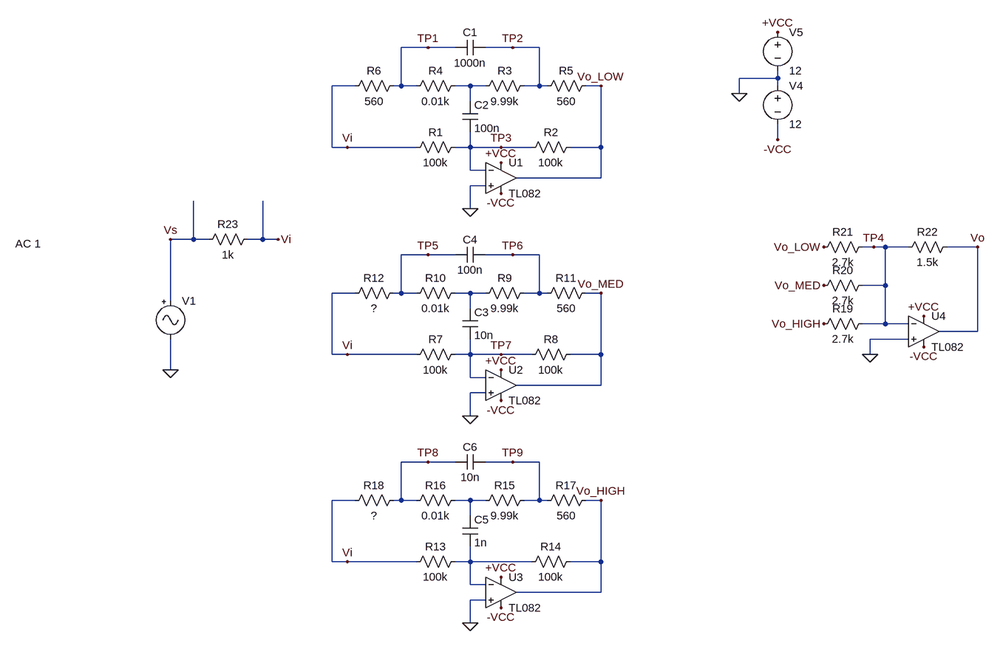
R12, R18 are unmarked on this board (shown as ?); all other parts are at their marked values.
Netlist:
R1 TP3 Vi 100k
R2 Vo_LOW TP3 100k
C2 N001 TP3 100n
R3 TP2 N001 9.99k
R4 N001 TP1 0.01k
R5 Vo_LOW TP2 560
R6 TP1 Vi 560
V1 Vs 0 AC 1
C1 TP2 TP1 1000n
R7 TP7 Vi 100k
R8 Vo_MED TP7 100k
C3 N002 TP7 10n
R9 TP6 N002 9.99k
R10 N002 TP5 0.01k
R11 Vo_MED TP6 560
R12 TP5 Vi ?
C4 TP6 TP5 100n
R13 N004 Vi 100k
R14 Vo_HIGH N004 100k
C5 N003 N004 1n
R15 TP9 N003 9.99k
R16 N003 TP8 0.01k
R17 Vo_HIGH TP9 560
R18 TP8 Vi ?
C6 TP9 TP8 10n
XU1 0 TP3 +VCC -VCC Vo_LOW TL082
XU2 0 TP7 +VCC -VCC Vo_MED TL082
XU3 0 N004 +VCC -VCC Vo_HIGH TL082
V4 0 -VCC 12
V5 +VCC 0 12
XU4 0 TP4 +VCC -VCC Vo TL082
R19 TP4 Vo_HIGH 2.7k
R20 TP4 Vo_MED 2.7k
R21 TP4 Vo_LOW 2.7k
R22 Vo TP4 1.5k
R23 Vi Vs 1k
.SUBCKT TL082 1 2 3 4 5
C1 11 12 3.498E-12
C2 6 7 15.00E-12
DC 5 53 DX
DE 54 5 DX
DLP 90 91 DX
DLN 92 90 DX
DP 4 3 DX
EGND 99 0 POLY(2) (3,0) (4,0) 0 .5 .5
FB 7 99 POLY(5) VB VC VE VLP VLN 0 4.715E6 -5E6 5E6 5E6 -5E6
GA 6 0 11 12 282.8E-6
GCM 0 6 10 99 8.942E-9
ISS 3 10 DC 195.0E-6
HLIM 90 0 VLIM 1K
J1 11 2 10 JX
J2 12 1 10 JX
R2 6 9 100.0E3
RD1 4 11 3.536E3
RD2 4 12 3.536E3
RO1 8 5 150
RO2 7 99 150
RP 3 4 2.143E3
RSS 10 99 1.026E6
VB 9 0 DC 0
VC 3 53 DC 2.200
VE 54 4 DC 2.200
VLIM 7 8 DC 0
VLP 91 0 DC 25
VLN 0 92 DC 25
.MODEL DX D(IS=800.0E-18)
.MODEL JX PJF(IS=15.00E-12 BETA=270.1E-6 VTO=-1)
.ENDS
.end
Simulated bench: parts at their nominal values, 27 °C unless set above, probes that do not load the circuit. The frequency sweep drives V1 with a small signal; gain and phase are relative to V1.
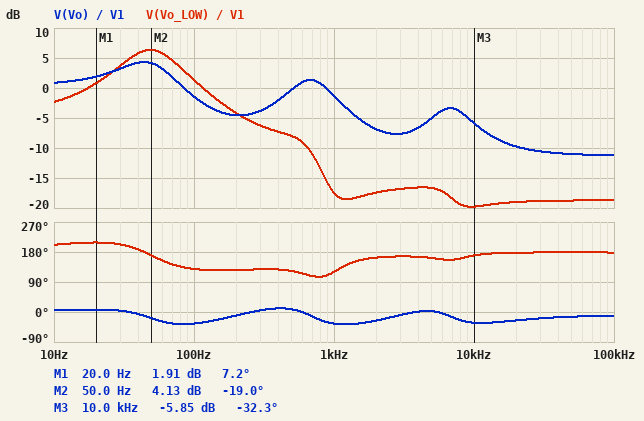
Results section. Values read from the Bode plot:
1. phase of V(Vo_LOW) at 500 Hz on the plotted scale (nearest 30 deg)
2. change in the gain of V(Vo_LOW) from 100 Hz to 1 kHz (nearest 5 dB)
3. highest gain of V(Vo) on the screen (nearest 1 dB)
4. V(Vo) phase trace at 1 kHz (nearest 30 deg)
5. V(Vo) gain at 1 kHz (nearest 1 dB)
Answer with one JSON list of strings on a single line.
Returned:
["120 deg", "-20 dB", "4 dB", "-30 deg", "-1 dB"]
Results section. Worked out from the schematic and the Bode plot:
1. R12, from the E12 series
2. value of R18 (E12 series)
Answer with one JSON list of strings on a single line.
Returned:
["270 Ω", "470 Ω"]
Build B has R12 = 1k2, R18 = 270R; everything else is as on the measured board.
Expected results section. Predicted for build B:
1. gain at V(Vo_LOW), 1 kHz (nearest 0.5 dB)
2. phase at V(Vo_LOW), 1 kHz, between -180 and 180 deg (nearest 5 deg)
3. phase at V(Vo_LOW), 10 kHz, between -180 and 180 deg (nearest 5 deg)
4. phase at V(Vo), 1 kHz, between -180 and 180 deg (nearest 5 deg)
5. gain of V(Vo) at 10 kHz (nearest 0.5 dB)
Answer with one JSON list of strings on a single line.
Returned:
["-11.5 dB", "160 deg", "140 deg", "-25 deg", "-2.0 dB"]
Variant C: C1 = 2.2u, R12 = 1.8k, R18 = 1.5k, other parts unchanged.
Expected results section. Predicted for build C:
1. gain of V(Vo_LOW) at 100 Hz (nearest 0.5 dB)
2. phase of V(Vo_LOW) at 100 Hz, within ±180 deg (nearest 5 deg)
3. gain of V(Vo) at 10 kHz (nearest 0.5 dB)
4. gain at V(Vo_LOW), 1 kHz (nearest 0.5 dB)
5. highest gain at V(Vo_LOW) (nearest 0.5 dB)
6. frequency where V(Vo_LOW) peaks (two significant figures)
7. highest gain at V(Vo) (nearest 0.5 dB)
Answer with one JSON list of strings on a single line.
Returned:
["-4.5 dB", "135 deg", "-9.5 dB", "-11.0 dB", "2.5 dB", "32 Hz", "2.0 dB"]
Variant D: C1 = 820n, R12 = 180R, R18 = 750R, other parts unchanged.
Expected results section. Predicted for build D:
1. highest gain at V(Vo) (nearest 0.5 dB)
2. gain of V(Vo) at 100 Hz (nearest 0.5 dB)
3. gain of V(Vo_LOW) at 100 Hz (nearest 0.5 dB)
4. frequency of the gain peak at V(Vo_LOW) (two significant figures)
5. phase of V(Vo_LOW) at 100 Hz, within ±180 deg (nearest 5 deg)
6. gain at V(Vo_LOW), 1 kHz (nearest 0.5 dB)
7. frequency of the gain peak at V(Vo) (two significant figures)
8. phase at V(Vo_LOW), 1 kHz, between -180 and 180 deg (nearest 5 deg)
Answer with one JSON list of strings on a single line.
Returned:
["5.0 dB", "0 dB", "3.0 dB", "54 Hz", "130 deg", "-16.0 dB", "50 Hz", "95 deg"]
